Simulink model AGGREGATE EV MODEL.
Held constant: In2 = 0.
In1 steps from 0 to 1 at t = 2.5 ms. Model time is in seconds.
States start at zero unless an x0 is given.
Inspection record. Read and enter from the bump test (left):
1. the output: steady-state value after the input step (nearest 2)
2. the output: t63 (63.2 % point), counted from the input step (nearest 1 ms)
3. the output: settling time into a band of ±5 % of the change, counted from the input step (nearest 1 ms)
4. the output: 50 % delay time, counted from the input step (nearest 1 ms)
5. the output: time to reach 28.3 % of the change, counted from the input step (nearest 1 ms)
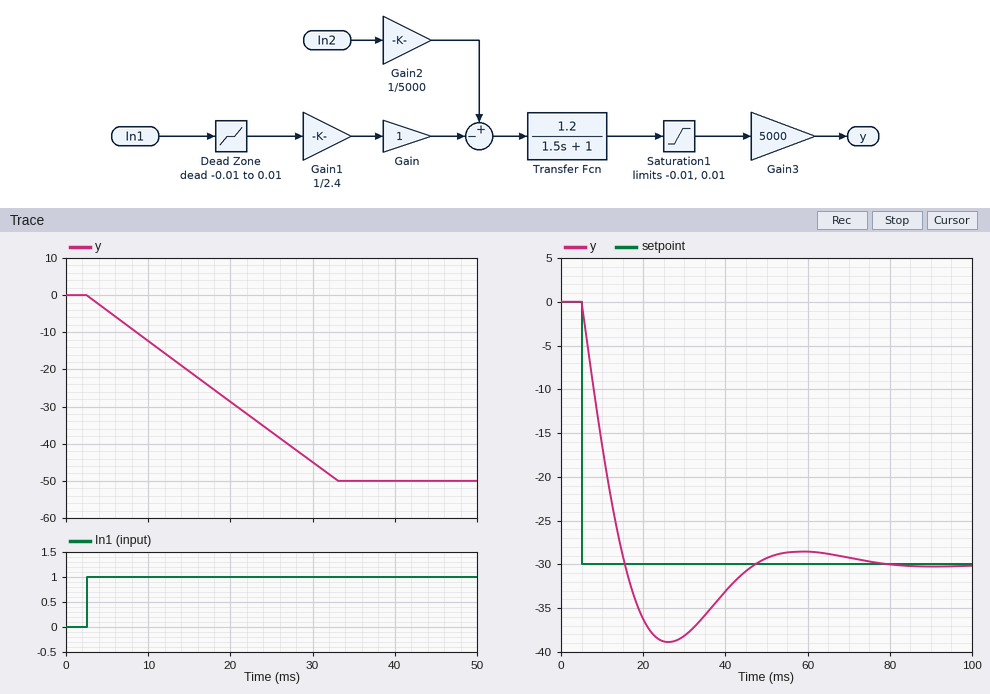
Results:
-50
19 ms
29 ms
15 ms
9 ms
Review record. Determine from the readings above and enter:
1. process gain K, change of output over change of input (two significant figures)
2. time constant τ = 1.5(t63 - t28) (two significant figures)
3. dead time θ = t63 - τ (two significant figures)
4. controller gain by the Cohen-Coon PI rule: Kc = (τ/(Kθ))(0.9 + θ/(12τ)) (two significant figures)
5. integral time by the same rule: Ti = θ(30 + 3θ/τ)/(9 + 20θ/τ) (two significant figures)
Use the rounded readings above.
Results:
-50
15 ms
4.0 ms
-0.069
8.6 ms
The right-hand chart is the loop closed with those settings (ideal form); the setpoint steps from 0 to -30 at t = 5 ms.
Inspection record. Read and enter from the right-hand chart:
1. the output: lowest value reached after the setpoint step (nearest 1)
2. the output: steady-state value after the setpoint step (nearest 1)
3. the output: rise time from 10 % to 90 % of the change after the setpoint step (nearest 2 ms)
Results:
-39
-30
8 ms
